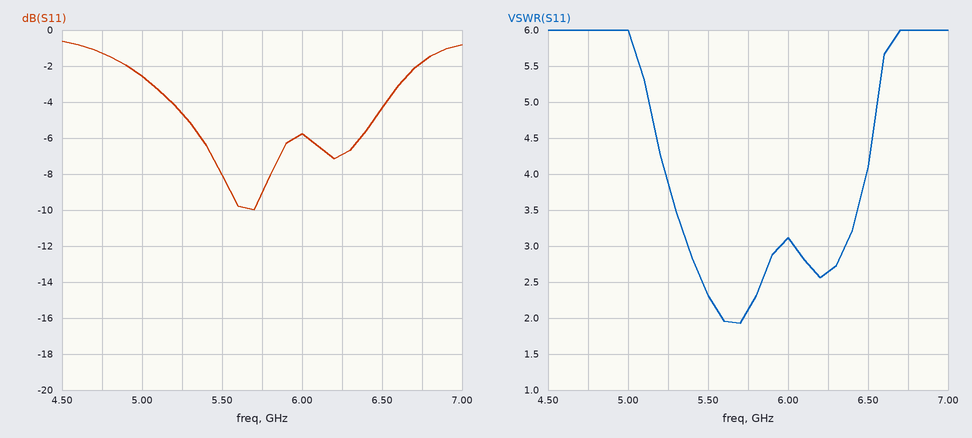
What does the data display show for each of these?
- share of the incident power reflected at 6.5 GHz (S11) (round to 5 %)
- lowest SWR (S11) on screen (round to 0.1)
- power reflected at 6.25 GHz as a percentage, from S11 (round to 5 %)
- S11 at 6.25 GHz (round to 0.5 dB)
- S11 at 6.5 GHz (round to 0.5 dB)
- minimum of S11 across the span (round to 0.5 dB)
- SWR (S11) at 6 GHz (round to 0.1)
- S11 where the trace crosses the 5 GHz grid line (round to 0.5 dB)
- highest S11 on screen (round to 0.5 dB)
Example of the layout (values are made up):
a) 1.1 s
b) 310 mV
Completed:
a) 35 %
b) 1.9
c) 20 %
d) -7.0 dB
e) -4.5 dB
f) -10.0 dB
g) 3.1
h) -2.5 dB
i) -0.5 dB
